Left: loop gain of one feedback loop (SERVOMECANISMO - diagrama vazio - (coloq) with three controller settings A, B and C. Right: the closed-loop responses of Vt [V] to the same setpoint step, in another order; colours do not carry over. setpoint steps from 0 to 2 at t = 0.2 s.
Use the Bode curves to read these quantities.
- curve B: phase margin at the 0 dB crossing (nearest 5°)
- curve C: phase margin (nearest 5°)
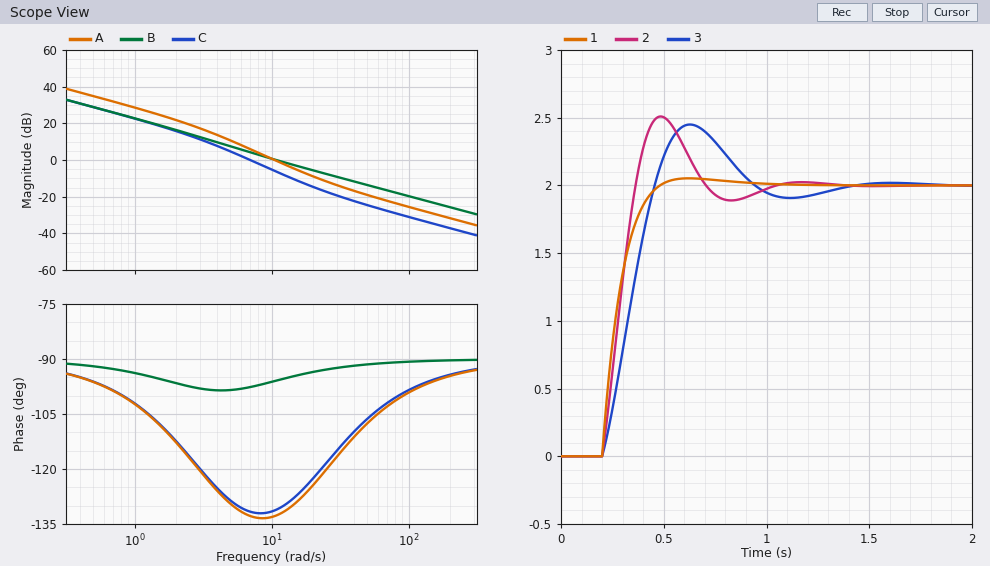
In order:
85°
50°
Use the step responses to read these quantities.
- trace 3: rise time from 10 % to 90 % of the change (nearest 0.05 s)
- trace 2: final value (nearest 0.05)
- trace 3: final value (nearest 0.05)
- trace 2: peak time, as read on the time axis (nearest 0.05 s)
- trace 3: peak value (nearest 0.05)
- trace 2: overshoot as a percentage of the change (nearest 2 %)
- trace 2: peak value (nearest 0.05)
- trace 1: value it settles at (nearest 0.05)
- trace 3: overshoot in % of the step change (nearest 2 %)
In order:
0.20 s
2.00
2.00
0.50 s
2.45
26 %
2.50
2.00
22 %
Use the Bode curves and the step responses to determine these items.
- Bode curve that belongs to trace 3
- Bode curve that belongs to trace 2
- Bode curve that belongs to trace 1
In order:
C
A
B
